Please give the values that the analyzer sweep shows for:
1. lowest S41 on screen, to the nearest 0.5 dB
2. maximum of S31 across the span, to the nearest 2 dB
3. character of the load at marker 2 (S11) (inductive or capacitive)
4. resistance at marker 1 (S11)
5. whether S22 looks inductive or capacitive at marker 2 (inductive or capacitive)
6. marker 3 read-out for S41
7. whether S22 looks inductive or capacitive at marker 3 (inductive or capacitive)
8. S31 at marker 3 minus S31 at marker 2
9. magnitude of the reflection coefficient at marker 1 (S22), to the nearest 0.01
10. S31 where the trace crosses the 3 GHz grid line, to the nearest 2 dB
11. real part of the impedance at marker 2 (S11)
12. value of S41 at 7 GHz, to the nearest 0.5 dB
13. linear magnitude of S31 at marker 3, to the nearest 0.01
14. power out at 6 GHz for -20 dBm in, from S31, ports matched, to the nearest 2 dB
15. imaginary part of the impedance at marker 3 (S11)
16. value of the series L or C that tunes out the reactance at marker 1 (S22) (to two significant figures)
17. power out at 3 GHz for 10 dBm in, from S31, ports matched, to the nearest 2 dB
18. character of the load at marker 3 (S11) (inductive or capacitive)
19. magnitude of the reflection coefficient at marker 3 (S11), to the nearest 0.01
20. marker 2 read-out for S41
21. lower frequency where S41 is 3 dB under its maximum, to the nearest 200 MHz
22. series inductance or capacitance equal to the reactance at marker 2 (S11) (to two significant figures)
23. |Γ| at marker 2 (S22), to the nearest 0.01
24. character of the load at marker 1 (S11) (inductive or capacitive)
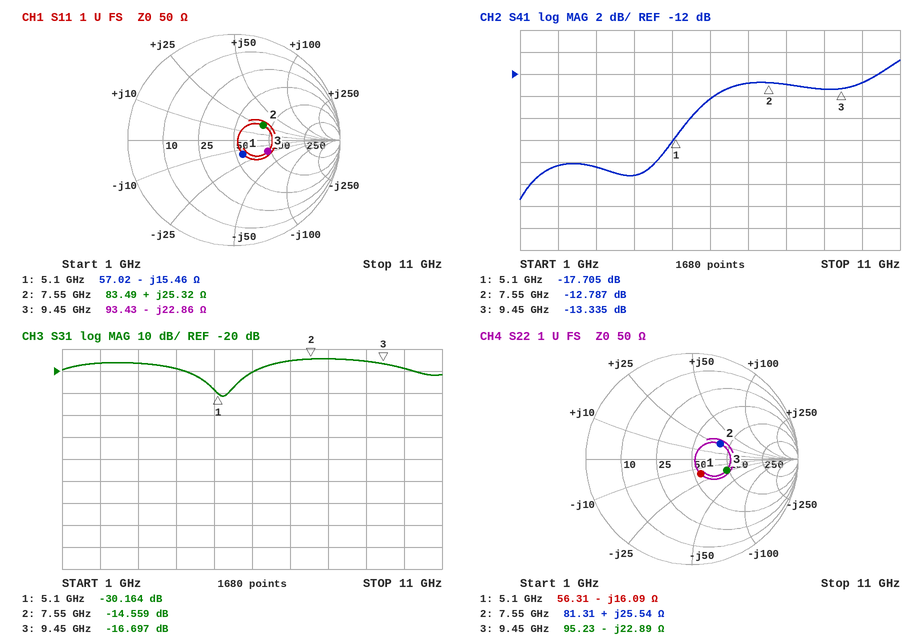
-23.5 dB
-14 dB
inductive
57.02 Ω
inductive
-13.335 dB
capacitive
-2.138 dB
0.16
-16 dB
83.49 Ω
-13.0 dB
0.15
-40 dBm
-22.86 Ω
500 pH
-6 dBm
capacitive
0.34
-12.787 dB
6.2 GHz
530 pH
0.30
capacitive
